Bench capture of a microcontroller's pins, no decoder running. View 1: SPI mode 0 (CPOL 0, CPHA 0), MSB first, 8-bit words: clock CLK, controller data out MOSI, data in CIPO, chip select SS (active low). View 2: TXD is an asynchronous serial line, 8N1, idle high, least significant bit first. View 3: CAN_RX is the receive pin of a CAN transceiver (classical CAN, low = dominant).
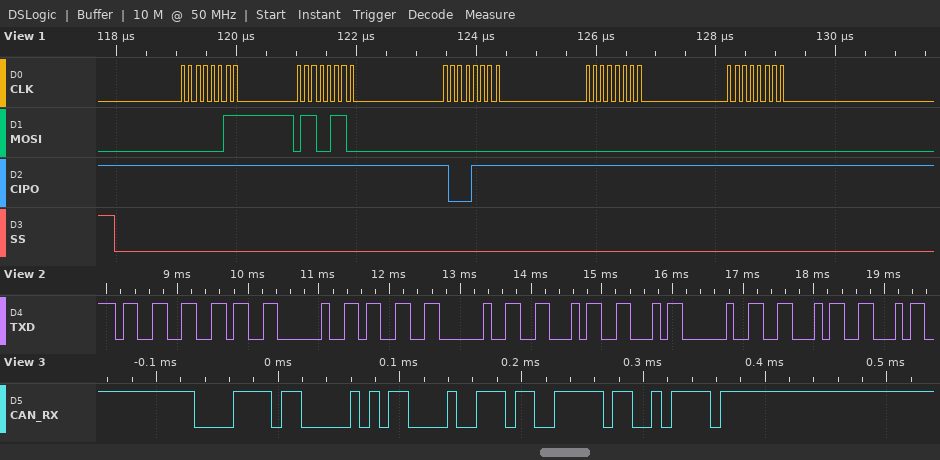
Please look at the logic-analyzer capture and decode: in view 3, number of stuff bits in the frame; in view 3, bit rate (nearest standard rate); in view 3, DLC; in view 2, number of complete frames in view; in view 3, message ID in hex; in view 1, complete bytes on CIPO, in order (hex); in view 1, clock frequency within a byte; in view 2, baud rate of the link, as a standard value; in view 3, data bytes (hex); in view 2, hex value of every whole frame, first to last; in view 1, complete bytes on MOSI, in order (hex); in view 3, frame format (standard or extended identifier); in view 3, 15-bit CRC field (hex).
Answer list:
2
125 kbit/s
2
10
0x0F6
FF FF 8F FF FF
8 MHz
9600 baud
C2 76
33 36 20 33 20 46 46 20 46 46
03 66 00 00 00
standard
0x3F97
